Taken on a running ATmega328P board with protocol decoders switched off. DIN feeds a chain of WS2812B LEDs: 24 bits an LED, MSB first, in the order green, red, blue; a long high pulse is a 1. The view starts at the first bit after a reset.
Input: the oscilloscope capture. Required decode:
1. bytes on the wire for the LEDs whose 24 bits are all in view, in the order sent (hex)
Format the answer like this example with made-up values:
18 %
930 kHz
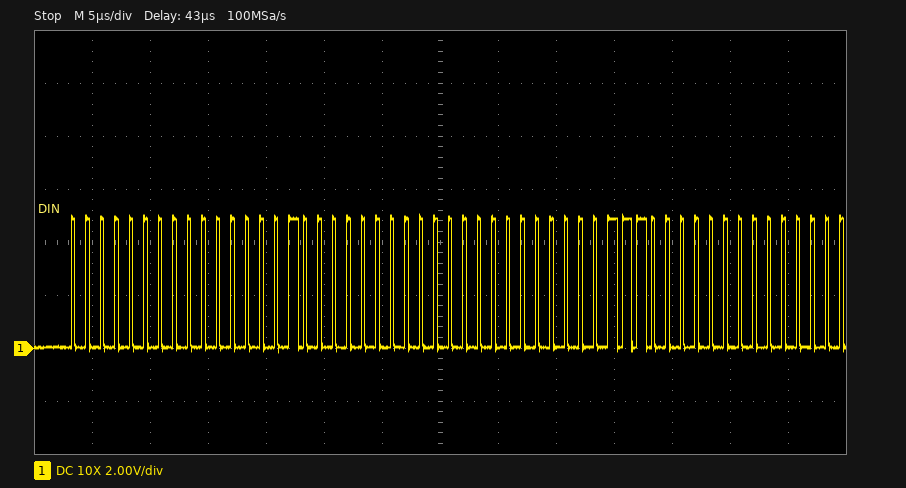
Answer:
00 01 00 00 07 00
